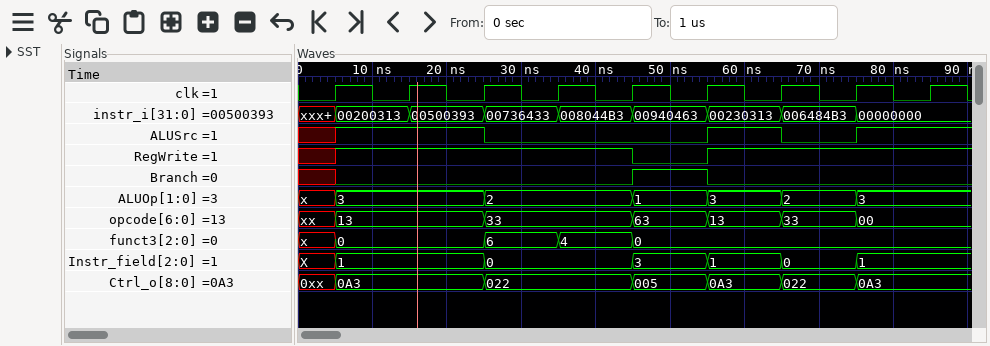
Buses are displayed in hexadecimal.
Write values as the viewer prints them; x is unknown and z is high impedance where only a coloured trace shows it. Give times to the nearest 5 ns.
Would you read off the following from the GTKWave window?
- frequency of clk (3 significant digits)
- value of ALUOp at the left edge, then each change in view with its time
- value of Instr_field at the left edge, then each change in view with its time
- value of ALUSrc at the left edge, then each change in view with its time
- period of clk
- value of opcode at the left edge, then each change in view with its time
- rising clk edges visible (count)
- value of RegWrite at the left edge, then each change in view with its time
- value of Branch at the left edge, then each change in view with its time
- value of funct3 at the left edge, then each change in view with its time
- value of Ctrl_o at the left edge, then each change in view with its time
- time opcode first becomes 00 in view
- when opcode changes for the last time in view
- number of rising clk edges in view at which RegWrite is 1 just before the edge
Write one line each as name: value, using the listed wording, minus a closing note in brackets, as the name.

frequency of clk: 100 MHz
value of ALUOp at the left edge, then each change in view with its time: x, 3 at 5 ns, 2 at 25 ns, 1 at 45 ns, 3 at 55 ns, 2 at 65 ns, 3 at 75 ns
value of Instr_field at the left edge, then each change in view with its time: X, 1 at 5 ns, 0 at 25 ns, 3 at 45 ns, 1 at 55 ns, 0 at 65 ns, 1 at 75 ns
value of ALUSrc at the left edge, then each change in view with its time: x, 1 at 5 ns, 0 at 25 ns, 1 at 55 ns, 0 at 65 ns, 1 at 75 ns
period of clk: 10 ns
value of opcode at the left edge, then each change in view with its time: xx, 13 at 5 ns, 33 at 25 ns, 63 at 45 ns, 13 at 55 ns, 33 at 65 ns, 00 at 75 ns
rising clk edges visible: 9
value of RegWrite at the left edge, then each change in view with its time: x, 1 at 5 ns, 0 at 45 ns, 1 at 55 ns
value of Branch at the left edge, then each change in view with its time: x, 0 at 5 ns, 1 at 45 ns, 0 at 55 ns
value of funct3 at the left edge, then each change in view with its time: x, 0 at 5 ns, 6 at 25 ns, 4 at 35 ns, 0 at 45 ns
value of Ctrl_o at the left edge, then each change in view with its time: 0xx, 0A3 at 5 ns, 022 at 25 ns, 005 at 45 ns, 0A3 at 55 ns, 022 at 65 ns, 0A3 at 75 ns
time opcode first becomes 00 in view: 75 ns
when opcode changes for the last time in view: 75 ns
number of rising clk edges in view at which RegWrite is 1 just before the edge: 7
